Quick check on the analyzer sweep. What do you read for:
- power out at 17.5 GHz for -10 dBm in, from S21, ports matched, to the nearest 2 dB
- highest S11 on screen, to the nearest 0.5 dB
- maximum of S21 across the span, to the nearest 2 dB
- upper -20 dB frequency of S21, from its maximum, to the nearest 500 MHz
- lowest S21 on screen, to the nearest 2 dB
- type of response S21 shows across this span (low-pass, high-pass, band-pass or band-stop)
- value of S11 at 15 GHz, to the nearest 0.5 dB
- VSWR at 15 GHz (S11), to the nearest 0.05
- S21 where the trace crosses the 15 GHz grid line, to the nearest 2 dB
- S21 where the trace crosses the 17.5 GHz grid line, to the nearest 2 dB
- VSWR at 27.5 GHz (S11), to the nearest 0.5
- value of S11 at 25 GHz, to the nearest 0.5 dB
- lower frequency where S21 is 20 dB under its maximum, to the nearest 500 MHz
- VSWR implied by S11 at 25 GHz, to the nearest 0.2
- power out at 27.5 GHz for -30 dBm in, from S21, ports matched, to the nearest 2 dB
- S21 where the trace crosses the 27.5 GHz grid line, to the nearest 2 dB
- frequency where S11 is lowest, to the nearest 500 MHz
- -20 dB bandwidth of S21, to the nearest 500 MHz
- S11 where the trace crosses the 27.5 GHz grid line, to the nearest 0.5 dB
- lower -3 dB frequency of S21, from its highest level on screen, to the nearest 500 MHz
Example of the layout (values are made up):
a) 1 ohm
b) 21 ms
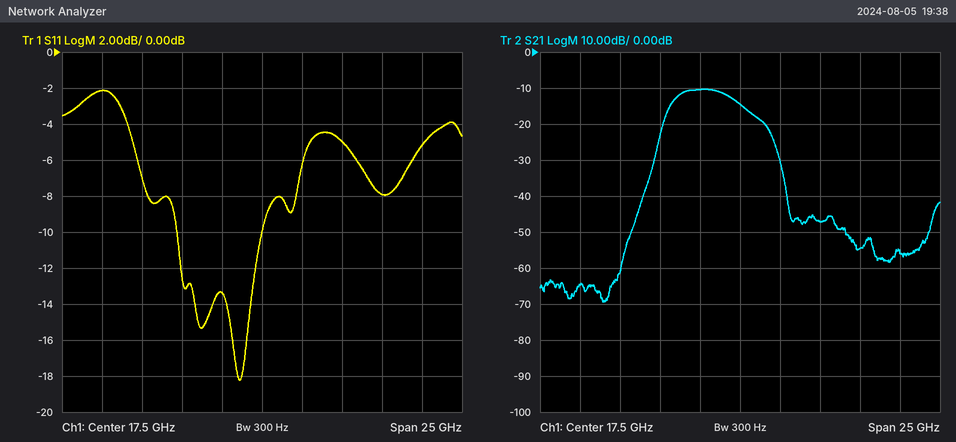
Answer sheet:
a) -24 dBm
b) -2.0 dB
c) -10 dB
d) 20.0 GHz
e) -70 dB
f) band-pass
g) -13.5 dB
h) 1.55
i) -10 dB
j) -14 dB
k) 3.5
l) -8.0 dB
m) 12.0 GHz
n) 2.4
o) -86 dBm
p) -56 dB
q) 16.0 GHz
r) 8.0 GHz
s) -5.0 dB
t) 13.5 GHz
